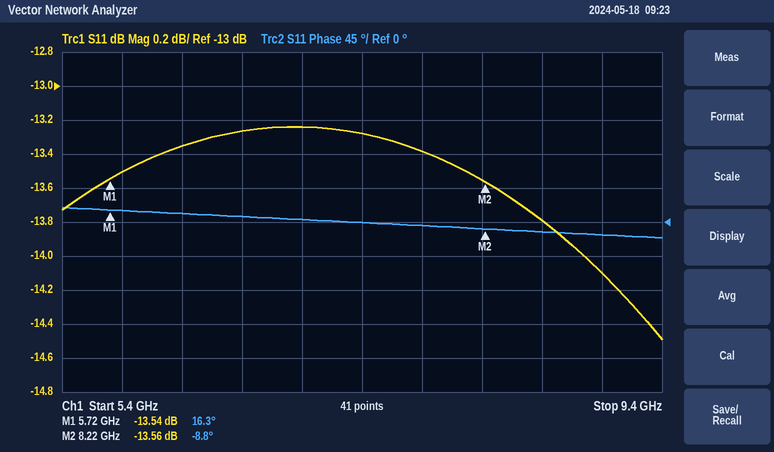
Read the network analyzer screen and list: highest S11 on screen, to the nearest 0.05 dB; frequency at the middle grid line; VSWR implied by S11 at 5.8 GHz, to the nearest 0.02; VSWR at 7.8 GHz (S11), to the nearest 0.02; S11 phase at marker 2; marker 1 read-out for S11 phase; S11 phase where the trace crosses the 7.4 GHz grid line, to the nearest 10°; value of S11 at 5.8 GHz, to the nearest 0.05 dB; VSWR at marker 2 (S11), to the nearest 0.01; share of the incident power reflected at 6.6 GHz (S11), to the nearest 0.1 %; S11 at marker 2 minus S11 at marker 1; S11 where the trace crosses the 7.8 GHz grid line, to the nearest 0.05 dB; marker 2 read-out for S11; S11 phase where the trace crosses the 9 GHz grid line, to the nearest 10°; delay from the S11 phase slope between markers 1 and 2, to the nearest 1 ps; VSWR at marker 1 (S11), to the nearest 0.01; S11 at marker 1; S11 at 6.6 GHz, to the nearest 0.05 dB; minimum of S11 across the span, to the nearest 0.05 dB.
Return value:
-13.25 dB
7.4 GHz
1.54
1.54
-8.8°
16.3°
0°
-13.50 dB
1.53
4.7 %
-0.02 dB
-13.40 dB
-13.56 dB
-20°
28 ps
1.53
-13.54 dB
-13.25 dB
-14.50 dB
